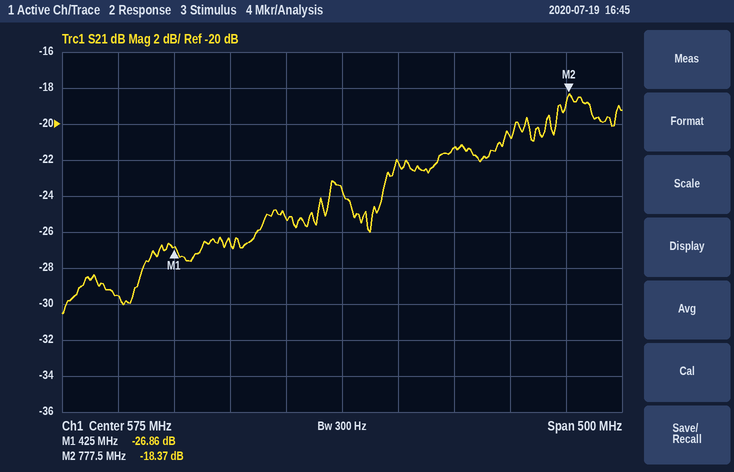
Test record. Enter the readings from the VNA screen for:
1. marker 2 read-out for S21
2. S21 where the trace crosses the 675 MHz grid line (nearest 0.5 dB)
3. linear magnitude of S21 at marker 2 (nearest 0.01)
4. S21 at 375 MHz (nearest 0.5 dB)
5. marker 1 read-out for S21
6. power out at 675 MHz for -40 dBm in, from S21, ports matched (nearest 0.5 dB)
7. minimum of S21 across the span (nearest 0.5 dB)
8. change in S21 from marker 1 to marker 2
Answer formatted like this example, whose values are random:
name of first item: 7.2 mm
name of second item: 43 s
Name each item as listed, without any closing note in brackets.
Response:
marker 2 read-out for S21: -18.37 dB
S21 where the trace crosses the 675 MHz grid line: -21.5 dB
linear magnitude of S21 at marker 2: 0.12
S21 at 375 MHz: -29.5 dB
marker 1 read-out for S21: -26.86 dB
power out at 675 MHz for -40 dBm in, from S21, ports matched: -61.5 dBm
minimum of S21 across the span: -30.5 dB
change in S21 from marker 1 to marker 2: 8.49 dB
